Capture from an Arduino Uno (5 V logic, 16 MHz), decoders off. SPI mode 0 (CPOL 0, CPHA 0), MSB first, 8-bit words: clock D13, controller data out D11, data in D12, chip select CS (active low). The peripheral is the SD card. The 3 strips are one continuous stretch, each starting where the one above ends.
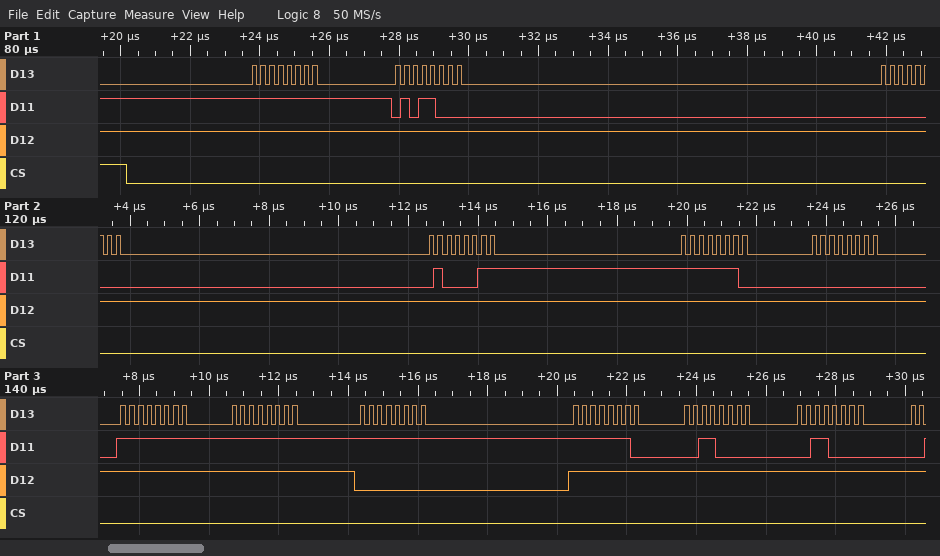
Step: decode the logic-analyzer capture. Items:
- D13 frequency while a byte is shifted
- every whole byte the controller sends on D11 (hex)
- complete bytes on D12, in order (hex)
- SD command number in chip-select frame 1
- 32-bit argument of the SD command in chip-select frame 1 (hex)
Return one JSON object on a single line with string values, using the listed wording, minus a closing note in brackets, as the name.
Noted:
{"D13 frequency while a byte is shifted": "4 MHz", "every whole byte the controller sends on D11": "FF 58 00 43 FE 00 FF FF FF FE 30 30", "complete bytes on D12, in order": "FF FF FF FF FF FF FF FF 00 FF FF FF", "SD command number in chip-select frame 1": "CMD24", "32-bit argument of the SD command in chip-select frame 1": "0x0043FE00"}
